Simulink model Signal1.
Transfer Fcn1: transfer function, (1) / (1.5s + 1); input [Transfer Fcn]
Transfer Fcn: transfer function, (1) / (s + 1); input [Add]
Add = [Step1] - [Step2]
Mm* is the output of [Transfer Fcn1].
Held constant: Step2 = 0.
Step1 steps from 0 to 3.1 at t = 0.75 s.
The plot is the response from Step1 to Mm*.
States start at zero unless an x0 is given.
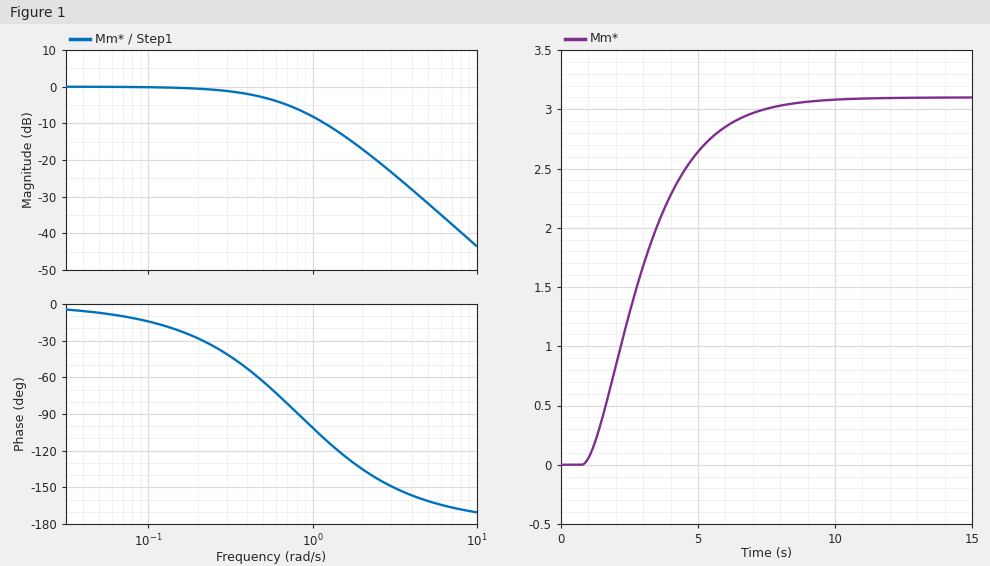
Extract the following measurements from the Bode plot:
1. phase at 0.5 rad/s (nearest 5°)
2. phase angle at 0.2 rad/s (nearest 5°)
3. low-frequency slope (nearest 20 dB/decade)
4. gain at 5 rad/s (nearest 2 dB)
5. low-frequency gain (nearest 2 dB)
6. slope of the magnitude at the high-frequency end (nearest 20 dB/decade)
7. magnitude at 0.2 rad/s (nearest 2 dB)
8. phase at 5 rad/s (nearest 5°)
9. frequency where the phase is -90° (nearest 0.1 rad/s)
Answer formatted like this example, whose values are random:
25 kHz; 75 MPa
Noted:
-65°; -30°; 0 dB/decade; -32 dB; 0 dB; -40 dB/decade; 0 dB; -160°; 0.8 rad/s
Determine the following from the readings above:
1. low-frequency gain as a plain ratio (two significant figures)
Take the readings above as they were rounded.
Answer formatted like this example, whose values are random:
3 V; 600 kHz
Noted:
1.0
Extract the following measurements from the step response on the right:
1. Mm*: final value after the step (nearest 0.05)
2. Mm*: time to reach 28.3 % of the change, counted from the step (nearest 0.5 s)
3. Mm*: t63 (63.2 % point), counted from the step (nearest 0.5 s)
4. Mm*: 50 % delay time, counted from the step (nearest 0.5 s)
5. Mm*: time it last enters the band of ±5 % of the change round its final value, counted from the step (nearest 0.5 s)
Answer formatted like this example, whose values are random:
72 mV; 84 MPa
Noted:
3.10; 1.5 s; 2.5 s; 2.0 s; 6.0 s
